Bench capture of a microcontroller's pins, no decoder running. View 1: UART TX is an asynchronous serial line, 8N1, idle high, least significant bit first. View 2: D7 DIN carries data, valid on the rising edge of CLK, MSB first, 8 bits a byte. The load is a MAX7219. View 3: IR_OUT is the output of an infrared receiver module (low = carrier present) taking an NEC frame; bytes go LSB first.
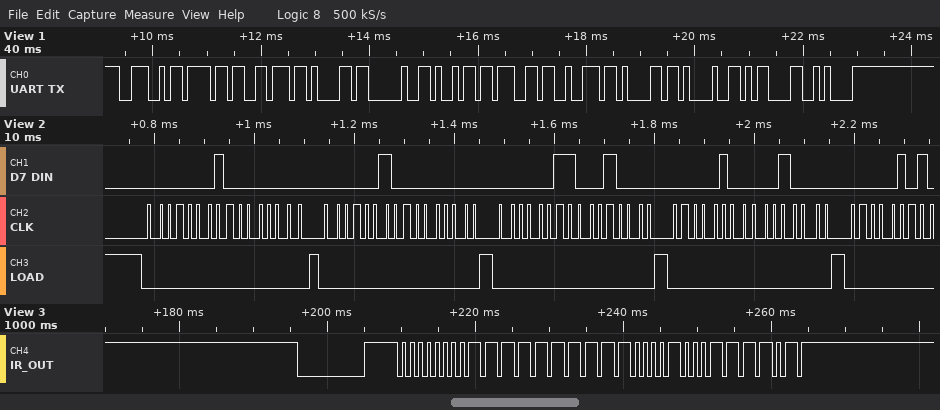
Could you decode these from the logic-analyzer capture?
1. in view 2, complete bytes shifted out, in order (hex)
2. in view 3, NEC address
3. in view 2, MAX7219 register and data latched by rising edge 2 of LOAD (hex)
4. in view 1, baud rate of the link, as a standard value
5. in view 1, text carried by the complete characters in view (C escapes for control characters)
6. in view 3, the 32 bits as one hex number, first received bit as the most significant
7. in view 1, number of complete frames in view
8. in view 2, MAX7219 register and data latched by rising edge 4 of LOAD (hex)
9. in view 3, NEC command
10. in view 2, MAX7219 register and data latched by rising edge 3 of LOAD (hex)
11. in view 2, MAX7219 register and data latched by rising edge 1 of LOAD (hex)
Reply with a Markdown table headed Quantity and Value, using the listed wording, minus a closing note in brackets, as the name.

| Quantity | Value |
|---|---|
| in view 2, complete bytes shifted out, in order | 01 00 02 00 03 10 04 10 05 |
| in view 3, NEC address | 0x00 |
| in view 2, MAX7219 register and data latched by rising edge 2 of LOAD | register 0x2, data 0x00 |
| in view 1, baud rate of the link, as a standard value | 9600 baud |
| in view 1, text carried by the complete characters in view | "Nova igra!\r\n" |
| in view 3, the 32 bits as one hex number, first received bit as the most significant | 0x00FFC23D |
| in view 1, number of complete frames in view | 12 |
| in view 2, MAX7219 register and data latched by rising edge 4 of LOAD | register 0x4, data 0x10 |
| in view 3, NEC command | 0x43 |
| in view 2, MAX7219 register and data latched by rising edge 3 of LOAD | register 0x3, data 0x10 |
| in view 2, MAX7219 register and data latched by rising edge 1 of LOAD | register 0x1, data 0x00 |
